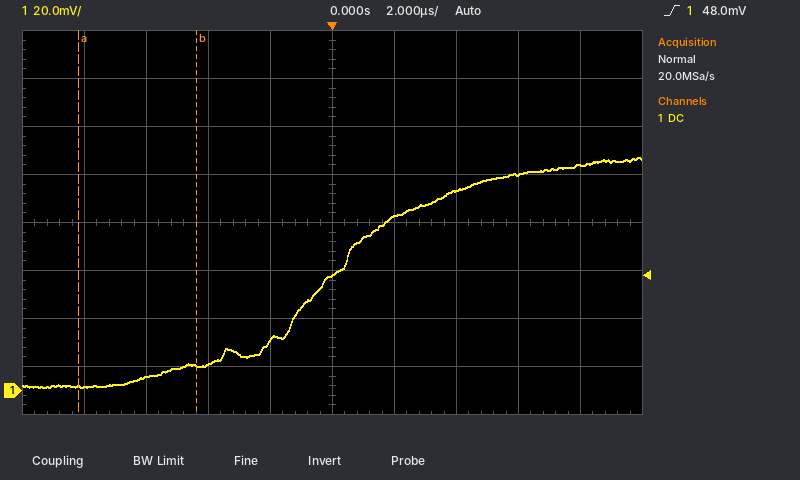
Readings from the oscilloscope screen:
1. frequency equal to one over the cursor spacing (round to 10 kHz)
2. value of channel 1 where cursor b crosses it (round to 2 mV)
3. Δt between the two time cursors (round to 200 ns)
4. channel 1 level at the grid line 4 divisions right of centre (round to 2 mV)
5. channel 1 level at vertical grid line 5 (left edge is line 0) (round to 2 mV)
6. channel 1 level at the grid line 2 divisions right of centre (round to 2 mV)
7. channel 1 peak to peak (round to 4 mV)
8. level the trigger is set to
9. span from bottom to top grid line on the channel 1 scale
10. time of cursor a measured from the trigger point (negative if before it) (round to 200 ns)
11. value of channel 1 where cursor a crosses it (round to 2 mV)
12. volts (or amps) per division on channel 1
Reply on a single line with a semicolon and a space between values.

260 kHz; 10 mV; 3.8 µs; 94 mV; 48 mV; 84 mV; 96 mV; 48.0 mV; 160 mV; -8.2 µs; 2 mV; 20 mV
